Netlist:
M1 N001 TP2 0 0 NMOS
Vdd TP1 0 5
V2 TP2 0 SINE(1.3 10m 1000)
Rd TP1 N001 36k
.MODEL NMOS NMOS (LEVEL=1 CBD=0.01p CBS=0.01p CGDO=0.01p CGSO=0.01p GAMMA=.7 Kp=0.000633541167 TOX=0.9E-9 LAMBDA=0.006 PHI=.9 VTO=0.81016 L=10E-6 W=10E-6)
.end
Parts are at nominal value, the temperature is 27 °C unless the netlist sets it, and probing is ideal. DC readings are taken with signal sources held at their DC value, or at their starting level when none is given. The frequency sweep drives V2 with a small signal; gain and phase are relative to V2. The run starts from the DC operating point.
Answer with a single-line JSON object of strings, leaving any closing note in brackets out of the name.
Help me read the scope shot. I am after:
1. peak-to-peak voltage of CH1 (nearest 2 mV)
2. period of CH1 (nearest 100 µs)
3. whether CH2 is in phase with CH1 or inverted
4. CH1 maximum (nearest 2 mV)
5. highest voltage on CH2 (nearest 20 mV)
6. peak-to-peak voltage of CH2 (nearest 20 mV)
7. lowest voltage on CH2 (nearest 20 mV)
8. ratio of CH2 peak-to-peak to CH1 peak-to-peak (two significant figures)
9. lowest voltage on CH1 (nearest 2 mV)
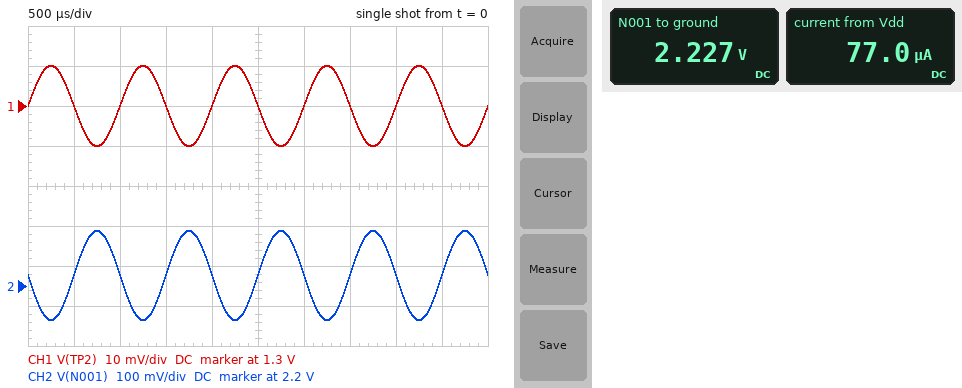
{"peak-to-peak voltage of CH1": "20 mV", "period of CH1": "1.0 ms", "whether CH2 is in phase with CH1 or inverted": "inverted", "CH1 maximum": "1.310 V", "highest voltage on CH2": "2.34 V", "peak-to-peak voltage of CH2": "220 mV", "lowest voltage on CH2": "2.12 V", "ratio of CH2 peak-to-peak to CH1 peak-to-peak": "11", "lowest voltage on CH1": "1.290 V"}
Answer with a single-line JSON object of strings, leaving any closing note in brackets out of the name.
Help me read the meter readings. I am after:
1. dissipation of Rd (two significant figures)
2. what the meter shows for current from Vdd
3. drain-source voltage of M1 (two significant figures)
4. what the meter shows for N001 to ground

{"dissipation of Rd": "210 µW", "what the meter shows for current from Vdd": "77.0 µA", "drain-source voltage of M1": "2.2 V", "what the meter shows for N001 to ground": "2.227 V"}
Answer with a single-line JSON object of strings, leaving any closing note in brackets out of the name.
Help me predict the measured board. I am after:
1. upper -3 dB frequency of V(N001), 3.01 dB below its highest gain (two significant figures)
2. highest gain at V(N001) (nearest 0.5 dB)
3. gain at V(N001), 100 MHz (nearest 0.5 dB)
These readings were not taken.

{"upper -3 dB frequency of V(N001), 3.01 dB below its highest gain": "870 MHz", "highest gain at V(N001)": "21.0 dB", "gain at V(N001), 100 MHz": "21.0 dB"}
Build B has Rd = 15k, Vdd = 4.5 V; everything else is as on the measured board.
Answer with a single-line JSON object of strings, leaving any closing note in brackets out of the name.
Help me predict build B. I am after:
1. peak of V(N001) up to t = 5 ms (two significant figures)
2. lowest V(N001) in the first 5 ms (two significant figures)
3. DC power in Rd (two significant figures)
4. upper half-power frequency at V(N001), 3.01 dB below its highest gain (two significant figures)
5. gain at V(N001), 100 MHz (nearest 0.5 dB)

{"peak of V(N001) up to t = 5 ms": "3.4 V", "lowest V(N001) in the first 5 ms": "3.3 V", "DC power in Rd": "90 µW", "upper half-power frequency at V(N001), 3.01 dB below its highest gain": "2.4 GHz", "gain at V(N001), 100 MHz": "13.5 dB"}
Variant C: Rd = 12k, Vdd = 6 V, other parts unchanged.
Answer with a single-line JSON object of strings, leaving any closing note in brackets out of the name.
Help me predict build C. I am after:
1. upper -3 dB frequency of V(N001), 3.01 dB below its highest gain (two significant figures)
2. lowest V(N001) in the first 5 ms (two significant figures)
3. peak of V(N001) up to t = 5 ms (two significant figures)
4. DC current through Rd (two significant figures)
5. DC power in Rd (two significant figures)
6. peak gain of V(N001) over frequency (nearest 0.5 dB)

{"upper -3 dB frequency of V(N001), 3.01 dB below its highest gain": "3.6 GHz", "lowest V(N001) in the first 5 ms": "5.0 V", "peak of V(N001) up to t = 5 ms": "5.1 V", "DC current through Rd": "78 µA", "DC power in Rd": "74 µW", "peak gain of V(N001) over frequency": "11.5 dB"}
